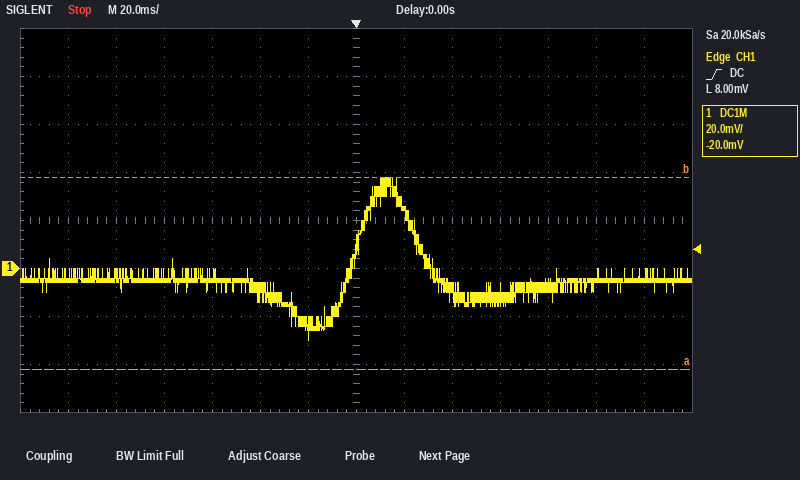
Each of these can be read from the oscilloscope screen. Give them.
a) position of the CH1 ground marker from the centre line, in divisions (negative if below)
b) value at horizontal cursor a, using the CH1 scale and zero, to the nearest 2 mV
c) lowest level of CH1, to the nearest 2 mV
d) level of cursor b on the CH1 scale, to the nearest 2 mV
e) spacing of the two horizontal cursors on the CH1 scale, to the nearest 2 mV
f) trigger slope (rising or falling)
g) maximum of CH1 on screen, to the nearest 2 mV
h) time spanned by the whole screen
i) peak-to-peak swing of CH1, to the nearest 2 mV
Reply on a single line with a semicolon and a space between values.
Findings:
-1.0 div; -42 mV; -30 mV; 38 mV; 80 mV; rising; 38 mV; 280 ms; 68 mV
